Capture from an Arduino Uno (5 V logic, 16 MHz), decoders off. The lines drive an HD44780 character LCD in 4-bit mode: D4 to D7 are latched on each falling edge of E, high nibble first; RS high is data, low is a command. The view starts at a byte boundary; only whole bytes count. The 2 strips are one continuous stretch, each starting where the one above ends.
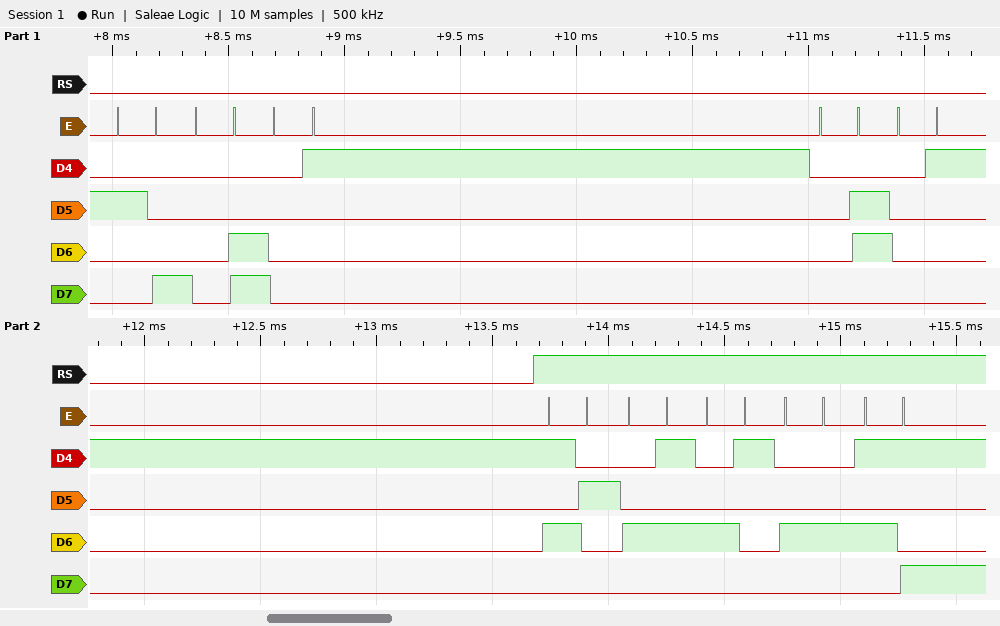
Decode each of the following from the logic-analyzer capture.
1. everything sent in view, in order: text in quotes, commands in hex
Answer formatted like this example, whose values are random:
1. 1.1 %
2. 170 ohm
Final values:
1. 0x28 0x0C 0x01 0x06 0x01 "READY"
